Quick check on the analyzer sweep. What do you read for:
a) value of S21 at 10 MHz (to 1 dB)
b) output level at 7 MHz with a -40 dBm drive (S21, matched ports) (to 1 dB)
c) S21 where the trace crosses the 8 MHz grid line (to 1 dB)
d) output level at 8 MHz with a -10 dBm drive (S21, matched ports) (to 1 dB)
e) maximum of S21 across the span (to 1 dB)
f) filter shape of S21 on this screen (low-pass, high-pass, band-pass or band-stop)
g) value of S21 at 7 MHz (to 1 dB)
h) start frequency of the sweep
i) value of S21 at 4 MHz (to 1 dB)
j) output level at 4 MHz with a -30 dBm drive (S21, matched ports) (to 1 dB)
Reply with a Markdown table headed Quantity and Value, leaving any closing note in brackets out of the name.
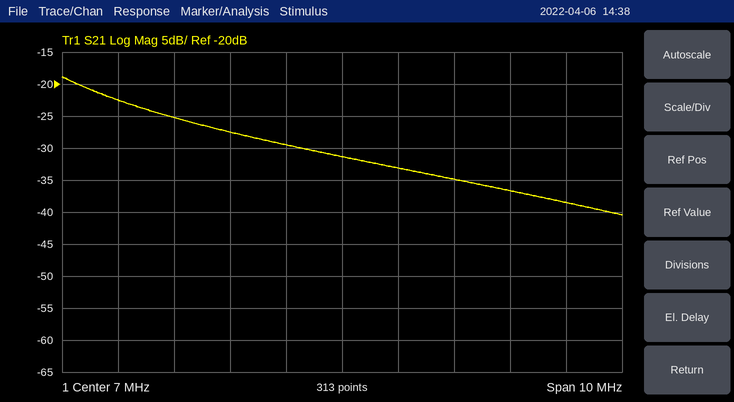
| Quantity | Value |
|---|---|
| value of S21 at 10 MHz | -37 dB |
| output level at 7 MHz with a -40 dBm drive (S21, matched ports) | -71 dBm |
| S21 where the trace crosses the 8 MHz grid line | -33 dB |
| output level at 8 MHz with a -10 dBm drive (S21, matched ports) | -43 dBm |
| maximum of S21 across the span | -19 dB |
| filter shape of S21 on this screen | low-pass |
| value of S21 at 7 MHz | -31 dB |
| start frequency of the sweep | 2 MHz |
| value of S21 at 4 MHz | -25 dB |
| output level at 4 MHz with a -30 dBm drive (S21, matched ports) | -55 dBm |
